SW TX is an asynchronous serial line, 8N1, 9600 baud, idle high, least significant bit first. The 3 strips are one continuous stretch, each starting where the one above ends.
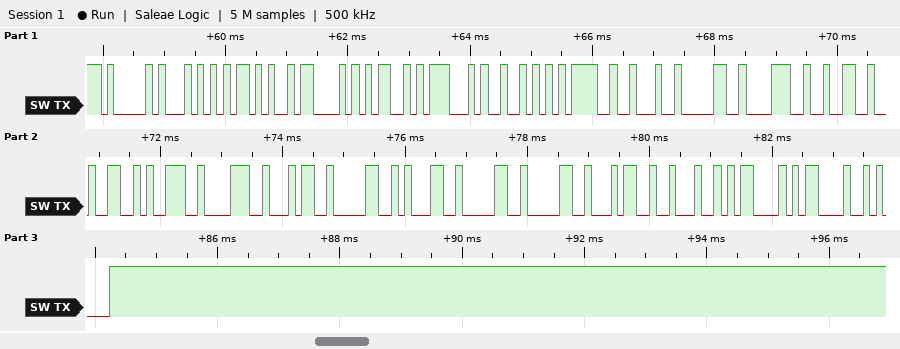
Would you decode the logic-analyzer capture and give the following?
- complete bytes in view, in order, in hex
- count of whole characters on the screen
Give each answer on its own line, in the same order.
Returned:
41 54 2B 43 4D 47 52 3D 22 30 38 32 32 39 38 34 30 31 30 30 34 22 0D 0D 0A
25
